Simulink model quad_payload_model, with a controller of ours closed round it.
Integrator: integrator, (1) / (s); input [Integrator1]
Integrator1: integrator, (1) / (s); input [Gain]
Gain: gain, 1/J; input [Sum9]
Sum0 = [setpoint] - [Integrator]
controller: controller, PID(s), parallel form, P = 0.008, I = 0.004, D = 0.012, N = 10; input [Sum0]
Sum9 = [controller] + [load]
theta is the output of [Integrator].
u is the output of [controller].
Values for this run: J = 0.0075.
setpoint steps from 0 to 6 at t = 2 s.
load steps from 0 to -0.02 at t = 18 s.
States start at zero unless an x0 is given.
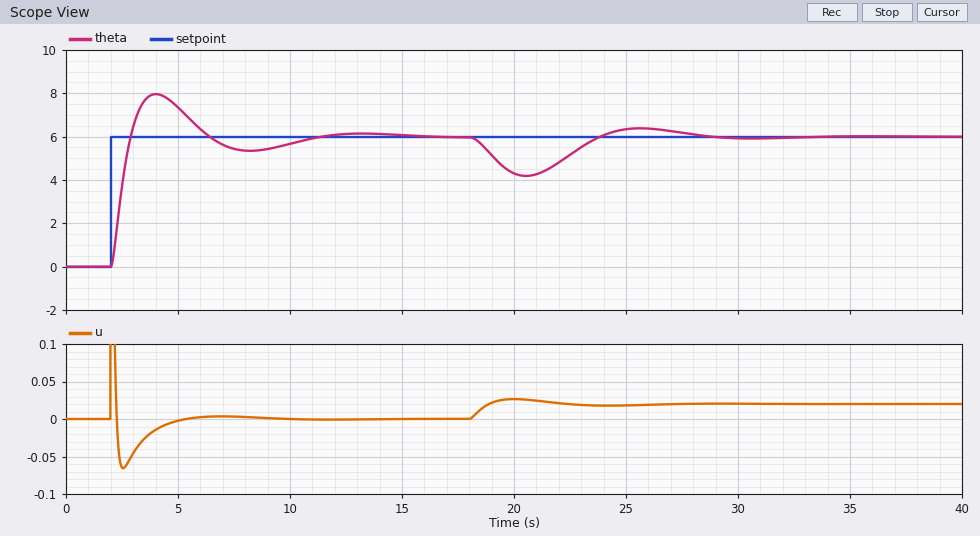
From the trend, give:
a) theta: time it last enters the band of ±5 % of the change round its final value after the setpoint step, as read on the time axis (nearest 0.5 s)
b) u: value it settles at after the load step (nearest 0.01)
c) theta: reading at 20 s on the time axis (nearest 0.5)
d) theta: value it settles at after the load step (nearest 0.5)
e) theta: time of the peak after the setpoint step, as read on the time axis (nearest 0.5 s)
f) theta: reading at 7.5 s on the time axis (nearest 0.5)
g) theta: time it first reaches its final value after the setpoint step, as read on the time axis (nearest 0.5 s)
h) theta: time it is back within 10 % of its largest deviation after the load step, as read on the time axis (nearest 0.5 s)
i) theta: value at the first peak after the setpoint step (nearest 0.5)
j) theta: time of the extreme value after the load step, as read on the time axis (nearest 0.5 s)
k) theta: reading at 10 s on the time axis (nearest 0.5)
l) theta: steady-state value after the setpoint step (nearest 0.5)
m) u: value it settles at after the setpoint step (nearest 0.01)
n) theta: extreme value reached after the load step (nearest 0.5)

10.0 s
0.02
4.5
6.0
4.0 s
5.5
3.0 s
27.5 s
8.0
20.5 s
5.5
6.0
0.00
4.0
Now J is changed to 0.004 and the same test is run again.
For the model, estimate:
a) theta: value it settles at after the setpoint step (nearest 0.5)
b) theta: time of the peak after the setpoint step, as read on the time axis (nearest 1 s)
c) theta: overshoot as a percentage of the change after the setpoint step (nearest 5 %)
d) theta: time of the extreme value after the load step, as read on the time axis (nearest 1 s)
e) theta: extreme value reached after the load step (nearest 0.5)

6.0
3 s
20 %
20 s
4.5
